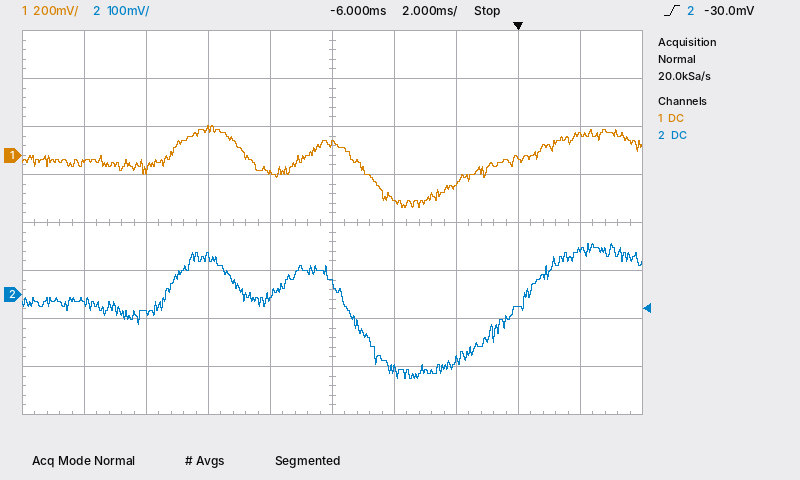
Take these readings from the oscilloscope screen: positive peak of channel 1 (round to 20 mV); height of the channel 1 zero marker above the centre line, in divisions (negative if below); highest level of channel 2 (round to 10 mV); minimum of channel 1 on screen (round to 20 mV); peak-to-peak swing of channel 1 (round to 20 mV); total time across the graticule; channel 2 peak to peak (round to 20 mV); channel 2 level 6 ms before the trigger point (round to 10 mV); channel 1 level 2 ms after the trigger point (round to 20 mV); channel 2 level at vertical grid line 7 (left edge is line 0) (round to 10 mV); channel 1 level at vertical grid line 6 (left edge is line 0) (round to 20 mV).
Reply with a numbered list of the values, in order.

1. 120 mV
2. +1.4 div
3. 110 mV
4. -220 mV
5. 340 mV
6. 20 ms
7. 280 mV
8. 20 mV
9. 80 mV
10. -140 mV
11. -180 mV
